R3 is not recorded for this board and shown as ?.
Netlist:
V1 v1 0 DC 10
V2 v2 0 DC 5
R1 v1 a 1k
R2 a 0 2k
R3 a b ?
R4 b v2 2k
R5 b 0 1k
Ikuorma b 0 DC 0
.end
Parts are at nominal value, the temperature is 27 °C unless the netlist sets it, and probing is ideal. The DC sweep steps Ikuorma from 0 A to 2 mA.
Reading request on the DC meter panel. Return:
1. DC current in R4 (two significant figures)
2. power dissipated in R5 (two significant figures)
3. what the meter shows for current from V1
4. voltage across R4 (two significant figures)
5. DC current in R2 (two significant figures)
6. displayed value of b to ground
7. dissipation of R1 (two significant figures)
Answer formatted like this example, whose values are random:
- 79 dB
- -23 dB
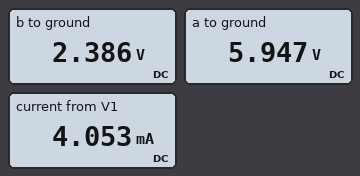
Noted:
- 1.3 mA
- 5.7 mW
- 4.053 mA
- 2.6 V
- 3.0 mA
- 2.386 V
- 16 mW
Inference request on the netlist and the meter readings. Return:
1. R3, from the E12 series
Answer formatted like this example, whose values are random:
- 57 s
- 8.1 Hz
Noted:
- 3.3 kΩ
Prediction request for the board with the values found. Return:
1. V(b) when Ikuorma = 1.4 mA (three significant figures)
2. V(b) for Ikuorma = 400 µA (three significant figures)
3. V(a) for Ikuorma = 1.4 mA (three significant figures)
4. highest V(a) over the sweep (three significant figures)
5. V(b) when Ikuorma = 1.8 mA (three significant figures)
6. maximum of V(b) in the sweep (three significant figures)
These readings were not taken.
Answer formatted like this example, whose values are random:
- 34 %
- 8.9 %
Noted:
- 1.59 V
- 2.16 V
- 5.81 V
- 5.95 V
- 1.36 V
- 2.39 V
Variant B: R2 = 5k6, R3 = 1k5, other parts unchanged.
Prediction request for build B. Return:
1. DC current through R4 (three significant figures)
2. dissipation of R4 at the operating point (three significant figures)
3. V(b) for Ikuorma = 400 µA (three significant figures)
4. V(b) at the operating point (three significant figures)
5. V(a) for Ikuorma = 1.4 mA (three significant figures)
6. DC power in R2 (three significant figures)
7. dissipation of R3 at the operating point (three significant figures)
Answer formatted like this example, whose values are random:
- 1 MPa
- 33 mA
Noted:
- 913 µA
- 1.67 mW
- 2.97 V
- 3.17 V
- 6.30 V
- 7.70 mW
- 7.67 mW
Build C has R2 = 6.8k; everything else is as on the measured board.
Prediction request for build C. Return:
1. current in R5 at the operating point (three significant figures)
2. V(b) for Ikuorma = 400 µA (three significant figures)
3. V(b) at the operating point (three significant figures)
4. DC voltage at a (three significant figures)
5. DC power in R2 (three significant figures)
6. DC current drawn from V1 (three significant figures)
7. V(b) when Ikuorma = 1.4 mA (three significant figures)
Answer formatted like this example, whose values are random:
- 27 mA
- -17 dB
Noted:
- 2.64 mA
- 2.41 V
- 2.64 V
- 7.45 V
- 8.16 mW
- 2.55 mA
- 1.83 V
